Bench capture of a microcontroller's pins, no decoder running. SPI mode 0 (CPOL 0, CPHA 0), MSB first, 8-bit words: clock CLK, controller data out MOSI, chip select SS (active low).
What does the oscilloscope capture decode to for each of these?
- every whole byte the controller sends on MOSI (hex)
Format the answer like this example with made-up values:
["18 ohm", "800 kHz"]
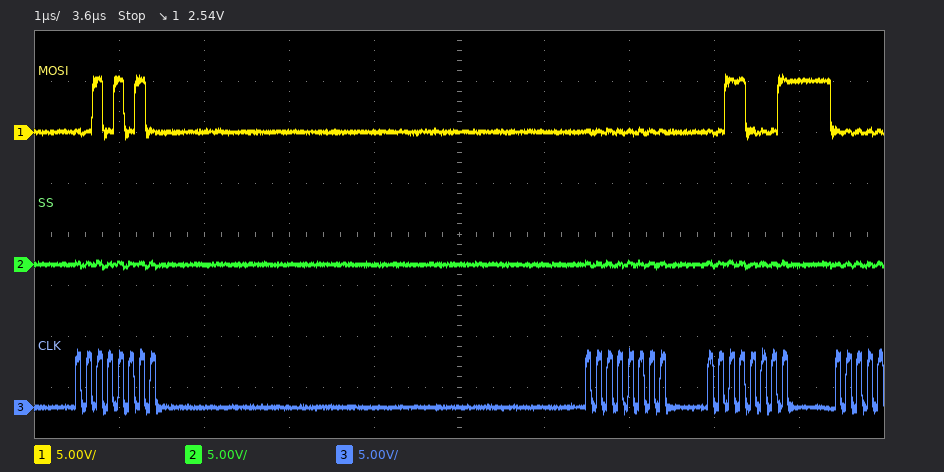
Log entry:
["2A 00 31"]
